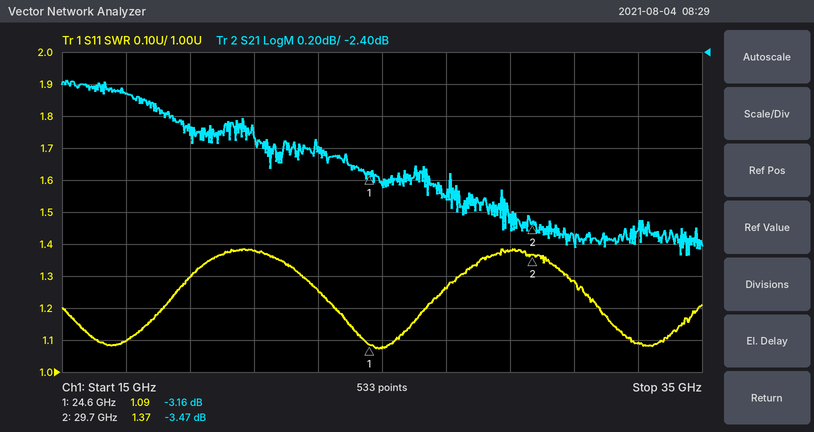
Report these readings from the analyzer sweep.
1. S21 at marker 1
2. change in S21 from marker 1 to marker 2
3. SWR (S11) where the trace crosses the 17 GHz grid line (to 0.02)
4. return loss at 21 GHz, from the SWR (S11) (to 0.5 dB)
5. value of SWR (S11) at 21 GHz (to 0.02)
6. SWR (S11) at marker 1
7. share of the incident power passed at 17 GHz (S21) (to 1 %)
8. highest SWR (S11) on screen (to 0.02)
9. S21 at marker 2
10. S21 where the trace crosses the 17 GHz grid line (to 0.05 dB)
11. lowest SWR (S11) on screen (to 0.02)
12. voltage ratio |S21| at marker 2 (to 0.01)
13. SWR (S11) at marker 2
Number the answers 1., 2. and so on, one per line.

1. -3.16 dB
2. -0.31 dB
3. 1.10
4. 16.0 dB
5. 1.38
6. 1.09
7. 54 %
8. 1.38
9. -3.47 dB
10. -2.65 dB
11. 1.08
12. 0.67
13. 1.37
